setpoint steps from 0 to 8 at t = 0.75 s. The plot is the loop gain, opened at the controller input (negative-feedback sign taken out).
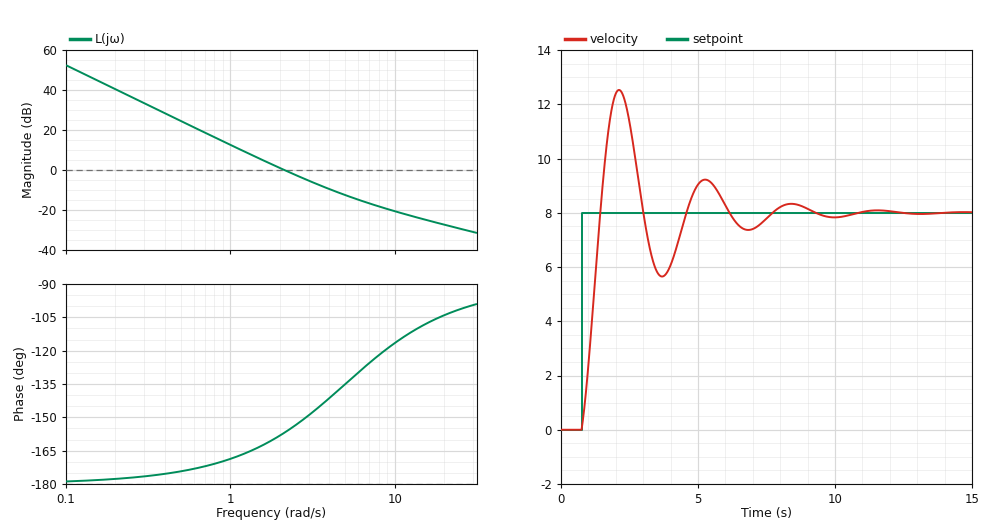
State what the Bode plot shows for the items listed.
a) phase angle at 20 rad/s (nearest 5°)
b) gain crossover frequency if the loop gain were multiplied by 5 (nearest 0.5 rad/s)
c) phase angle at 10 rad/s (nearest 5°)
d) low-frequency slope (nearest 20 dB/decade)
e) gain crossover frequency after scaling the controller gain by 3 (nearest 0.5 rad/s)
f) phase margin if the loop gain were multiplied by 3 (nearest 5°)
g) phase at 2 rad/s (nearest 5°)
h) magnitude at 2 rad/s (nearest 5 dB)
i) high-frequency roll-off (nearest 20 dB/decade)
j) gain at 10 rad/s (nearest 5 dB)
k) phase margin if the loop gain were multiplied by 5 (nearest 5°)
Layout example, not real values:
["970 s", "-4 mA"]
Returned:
["-105°", "5.5 rad/s", "-115°", "-40 dB/decade", "4.0 rad/s", "40°", "-160°", "0 dB", "-20 dB/decade", "-20 dB", "50°"]
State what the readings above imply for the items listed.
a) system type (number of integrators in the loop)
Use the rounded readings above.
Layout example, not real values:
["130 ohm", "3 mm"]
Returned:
["2"]
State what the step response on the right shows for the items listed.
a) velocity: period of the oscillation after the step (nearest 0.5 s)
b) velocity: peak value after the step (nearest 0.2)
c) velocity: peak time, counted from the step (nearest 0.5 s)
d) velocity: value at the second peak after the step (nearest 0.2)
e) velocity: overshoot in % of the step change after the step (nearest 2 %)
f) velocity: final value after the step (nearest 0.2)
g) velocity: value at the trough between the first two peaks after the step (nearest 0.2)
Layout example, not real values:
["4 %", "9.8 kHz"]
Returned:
["3.0 s", "12.6", "1.5 s", "9.2", "56 %", "8.0", "5.6"]
